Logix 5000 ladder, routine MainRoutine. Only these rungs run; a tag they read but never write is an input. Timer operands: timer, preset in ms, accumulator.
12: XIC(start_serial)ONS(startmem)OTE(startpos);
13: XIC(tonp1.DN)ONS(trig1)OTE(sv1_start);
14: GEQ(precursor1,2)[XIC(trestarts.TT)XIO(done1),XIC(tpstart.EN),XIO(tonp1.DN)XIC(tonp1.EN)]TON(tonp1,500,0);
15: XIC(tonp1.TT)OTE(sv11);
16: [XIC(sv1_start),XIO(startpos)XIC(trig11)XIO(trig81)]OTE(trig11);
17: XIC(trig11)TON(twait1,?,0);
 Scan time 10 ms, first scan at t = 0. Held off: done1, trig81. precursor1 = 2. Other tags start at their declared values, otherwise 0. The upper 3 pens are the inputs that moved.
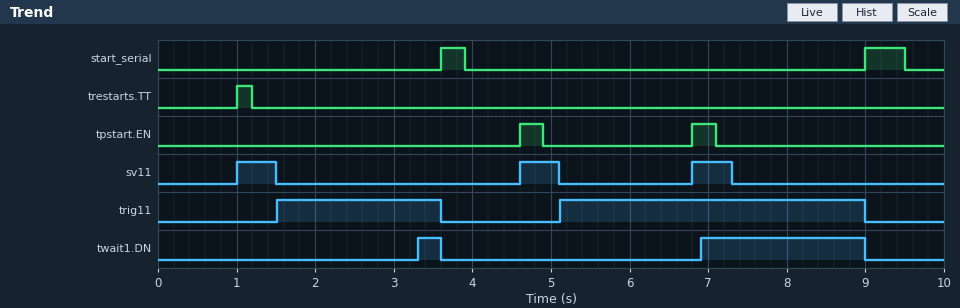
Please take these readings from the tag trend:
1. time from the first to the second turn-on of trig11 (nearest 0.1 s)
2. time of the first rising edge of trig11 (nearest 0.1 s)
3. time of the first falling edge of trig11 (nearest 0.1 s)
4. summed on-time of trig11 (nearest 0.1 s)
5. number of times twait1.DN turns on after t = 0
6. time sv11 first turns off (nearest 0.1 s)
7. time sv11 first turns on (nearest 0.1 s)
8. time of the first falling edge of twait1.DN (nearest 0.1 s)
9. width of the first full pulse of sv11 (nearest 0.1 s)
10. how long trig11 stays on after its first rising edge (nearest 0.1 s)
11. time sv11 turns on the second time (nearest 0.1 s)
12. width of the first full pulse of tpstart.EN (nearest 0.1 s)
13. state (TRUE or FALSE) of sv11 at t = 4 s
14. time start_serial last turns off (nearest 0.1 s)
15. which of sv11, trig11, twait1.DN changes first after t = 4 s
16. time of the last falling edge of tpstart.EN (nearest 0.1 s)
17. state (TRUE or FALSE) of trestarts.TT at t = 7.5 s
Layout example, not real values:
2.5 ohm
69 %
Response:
3.6 s
1.5 s
3.6 s
6.0 s
2
1.5 s
1.0 s
3.6 s
0.5 s
2.1 s
4.6 s
0.3 s
FALSE
9.5 s
sv11
7.1 s
FALSE
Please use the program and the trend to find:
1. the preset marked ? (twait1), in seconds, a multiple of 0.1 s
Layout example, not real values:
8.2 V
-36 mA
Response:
1.8 s
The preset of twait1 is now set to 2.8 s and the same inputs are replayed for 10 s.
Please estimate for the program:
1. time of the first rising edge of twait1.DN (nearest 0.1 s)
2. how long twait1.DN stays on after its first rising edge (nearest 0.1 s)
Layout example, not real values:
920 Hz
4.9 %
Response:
7.9 s
1.1 s
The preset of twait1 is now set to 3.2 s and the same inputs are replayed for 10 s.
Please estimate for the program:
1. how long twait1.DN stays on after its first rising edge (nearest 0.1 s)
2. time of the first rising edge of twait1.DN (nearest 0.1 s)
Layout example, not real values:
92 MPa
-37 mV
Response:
0.7 s
8.3 s
